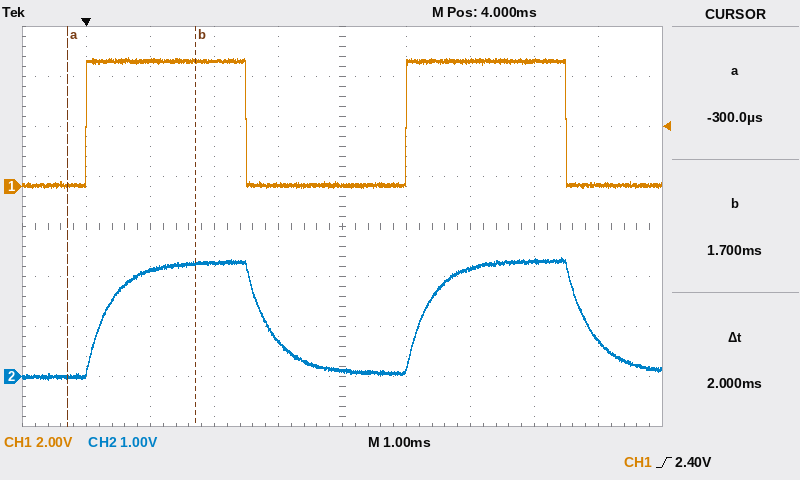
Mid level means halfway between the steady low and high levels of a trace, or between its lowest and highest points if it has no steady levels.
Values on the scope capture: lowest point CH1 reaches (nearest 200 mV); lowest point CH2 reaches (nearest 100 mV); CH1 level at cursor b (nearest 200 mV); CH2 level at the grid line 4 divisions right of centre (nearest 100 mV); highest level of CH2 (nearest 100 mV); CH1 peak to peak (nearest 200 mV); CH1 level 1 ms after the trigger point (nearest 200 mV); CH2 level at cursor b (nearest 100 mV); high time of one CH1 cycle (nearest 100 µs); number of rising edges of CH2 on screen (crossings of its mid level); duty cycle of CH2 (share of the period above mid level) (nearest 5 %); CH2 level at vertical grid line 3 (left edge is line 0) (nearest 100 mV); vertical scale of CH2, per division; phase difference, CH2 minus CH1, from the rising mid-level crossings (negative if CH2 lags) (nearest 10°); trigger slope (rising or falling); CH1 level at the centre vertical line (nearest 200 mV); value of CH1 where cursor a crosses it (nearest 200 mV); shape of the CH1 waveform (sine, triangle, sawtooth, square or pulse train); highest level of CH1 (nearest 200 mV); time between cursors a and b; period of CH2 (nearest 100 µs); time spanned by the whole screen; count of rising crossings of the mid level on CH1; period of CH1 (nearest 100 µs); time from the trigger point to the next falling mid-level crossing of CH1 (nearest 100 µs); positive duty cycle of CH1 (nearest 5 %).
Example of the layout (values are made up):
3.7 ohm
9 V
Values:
0.0 V
-100 mV
5.0 V
700 mV
2.4 V
5.2 V
5.0 V
2.3 V
2.5 ms
2
50 %
2.3 V
1 V
-20°
rising
0.0 V
0.0 V
square
5.2 V
2 ms
5.0 ms
10 ms
2
5.0 ms
2.5 ms
50 %
